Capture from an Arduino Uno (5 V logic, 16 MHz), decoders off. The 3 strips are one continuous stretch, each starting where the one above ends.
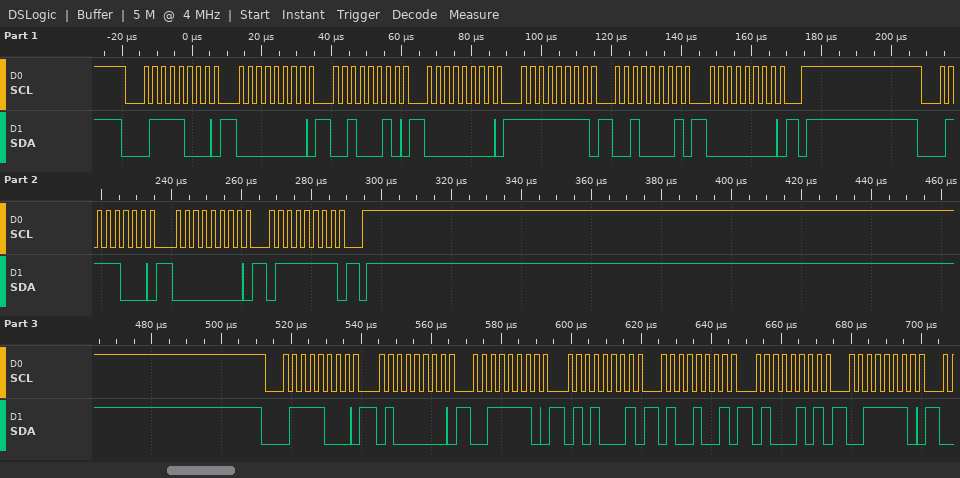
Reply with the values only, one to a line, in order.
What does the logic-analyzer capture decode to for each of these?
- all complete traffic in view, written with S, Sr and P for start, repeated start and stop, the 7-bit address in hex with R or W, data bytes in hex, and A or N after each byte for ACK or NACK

S 3CW A 00 A 22 A 00 A FF A 21 A 00 A P S 3CW A 00 A 7F A P S 3CW A 40 A 3E A 51 A 49 A 45 A 3E A
